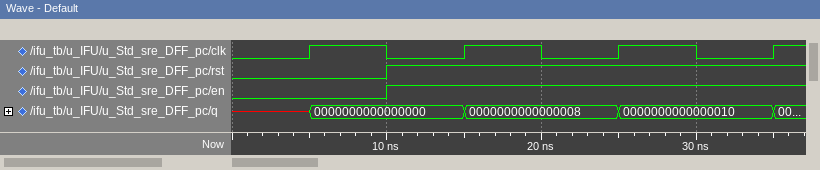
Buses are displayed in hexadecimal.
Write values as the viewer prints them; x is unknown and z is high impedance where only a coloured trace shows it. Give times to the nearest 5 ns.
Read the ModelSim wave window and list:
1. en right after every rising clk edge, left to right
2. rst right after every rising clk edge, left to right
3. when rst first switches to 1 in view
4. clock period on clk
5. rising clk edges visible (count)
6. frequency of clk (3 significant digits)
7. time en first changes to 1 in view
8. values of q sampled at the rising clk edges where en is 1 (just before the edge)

0 1 1 1
0 1 1 1
10 ns
10 ns
4
100 MHz
10 ns
0000000000000000, 0000000000000008, 0000000000000010
